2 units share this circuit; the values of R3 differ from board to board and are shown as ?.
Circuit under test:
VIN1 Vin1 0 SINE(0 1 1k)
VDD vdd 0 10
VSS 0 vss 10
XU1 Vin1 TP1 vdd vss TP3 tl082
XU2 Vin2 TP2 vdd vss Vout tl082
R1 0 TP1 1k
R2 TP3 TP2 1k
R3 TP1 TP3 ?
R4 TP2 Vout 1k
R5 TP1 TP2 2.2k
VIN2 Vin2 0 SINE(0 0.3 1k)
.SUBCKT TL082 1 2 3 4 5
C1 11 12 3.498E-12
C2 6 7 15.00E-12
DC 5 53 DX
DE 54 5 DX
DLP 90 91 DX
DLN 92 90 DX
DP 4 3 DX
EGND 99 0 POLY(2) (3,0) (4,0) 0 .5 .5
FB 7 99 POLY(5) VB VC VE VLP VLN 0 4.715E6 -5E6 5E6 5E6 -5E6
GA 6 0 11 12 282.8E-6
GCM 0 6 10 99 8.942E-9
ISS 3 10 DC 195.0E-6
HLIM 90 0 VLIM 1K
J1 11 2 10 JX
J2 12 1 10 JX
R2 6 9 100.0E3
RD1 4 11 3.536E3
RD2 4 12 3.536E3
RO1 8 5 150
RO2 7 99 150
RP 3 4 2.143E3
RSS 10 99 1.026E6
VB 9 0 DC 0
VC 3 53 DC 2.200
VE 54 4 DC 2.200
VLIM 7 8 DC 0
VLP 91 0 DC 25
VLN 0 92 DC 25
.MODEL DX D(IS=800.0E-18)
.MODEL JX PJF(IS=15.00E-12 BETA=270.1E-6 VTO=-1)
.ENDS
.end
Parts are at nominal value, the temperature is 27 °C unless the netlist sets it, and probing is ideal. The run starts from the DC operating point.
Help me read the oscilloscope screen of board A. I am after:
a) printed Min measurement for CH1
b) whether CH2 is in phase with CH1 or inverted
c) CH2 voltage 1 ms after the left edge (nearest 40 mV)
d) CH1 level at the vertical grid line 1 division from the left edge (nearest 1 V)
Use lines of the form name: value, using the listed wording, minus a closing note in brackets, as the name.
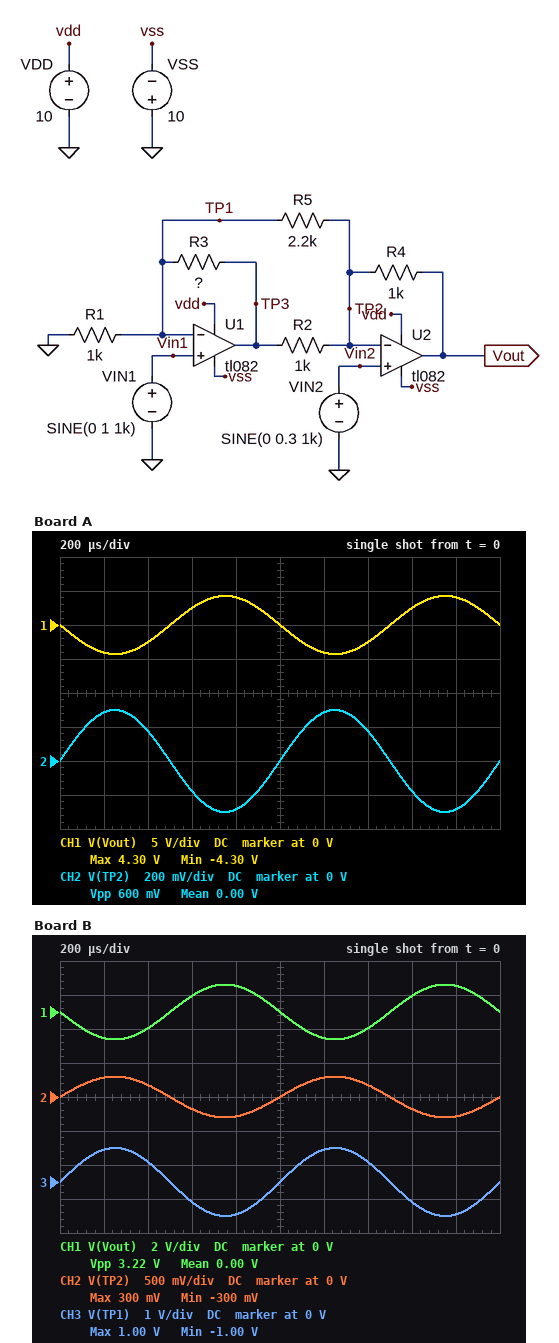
printed Min measurement for CH1: -4.30 V
whether CH2 is in phase with CH1 or inverted: inverted
CH2 voltage 1 ms after the left edge: 0 V
CH1 level at the vertical grid line 1 division from the left edge: -4 V
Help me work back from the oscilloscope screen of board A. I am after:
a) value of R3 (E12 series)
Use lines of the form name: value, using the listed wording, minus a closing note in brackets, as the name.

value of R3: 2.7 kΩ
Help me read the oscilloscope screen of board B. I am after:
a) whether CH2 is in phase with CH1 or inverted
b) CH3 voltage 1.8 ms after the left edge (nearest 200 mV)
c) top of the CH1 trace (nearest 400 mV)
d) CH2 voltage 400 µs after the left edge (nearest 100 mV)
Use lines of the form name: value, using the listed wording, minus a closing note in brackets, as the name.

whether CH2 is in phase with CH1 or inverted: inverted
CH3 voltage 1.8 ms after the left edge: -1.0 V
top of the CH1 trace: 1.6 V
CH2 voltage 400 µs after the left edge: 200 mV
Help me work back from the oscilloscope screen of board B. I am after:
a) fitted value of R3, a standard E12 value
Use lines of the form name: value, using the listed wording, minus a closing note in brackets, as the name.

fitted value of R3, a standard E12 value: 680 Ω
